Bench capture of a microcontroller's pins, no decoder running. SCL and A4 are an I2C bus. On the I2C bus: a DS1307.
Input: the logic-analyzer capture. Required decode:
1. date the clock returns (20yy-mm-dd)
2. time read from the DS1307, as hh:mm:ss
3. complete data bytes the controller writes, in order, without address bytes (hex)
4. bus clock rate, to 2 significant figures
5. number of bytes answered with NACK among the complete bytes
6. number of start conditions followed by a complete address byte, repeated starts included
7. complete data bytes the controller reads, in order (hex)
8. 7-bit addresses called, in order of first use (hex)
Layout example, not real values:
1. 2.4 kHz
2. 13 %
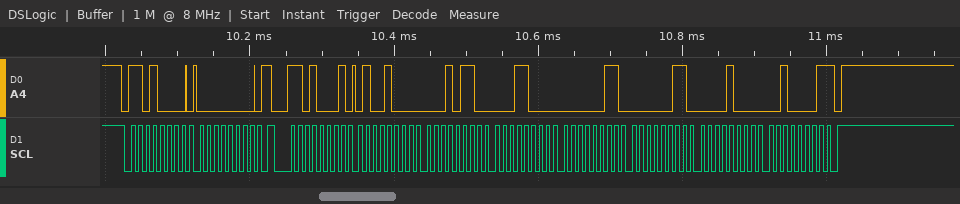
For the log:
1. 2021-08-03
2. 18:16:48
3. 00
4. 100 kHz
5. 1
6. 2
7. 48 16 18 03 03 08 21
8. 0x68
